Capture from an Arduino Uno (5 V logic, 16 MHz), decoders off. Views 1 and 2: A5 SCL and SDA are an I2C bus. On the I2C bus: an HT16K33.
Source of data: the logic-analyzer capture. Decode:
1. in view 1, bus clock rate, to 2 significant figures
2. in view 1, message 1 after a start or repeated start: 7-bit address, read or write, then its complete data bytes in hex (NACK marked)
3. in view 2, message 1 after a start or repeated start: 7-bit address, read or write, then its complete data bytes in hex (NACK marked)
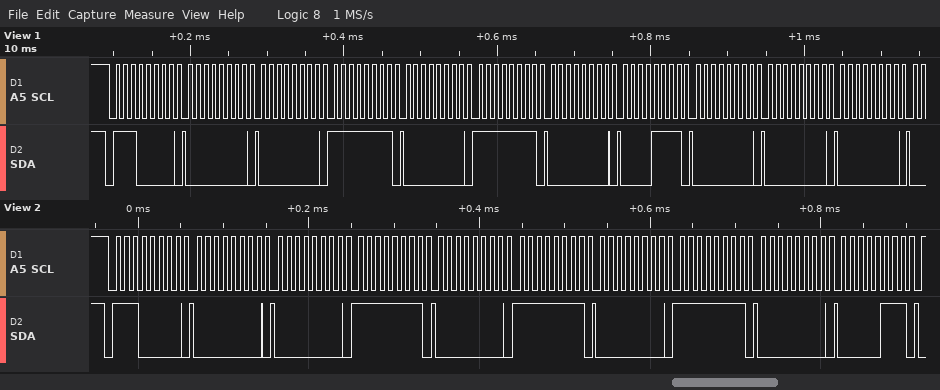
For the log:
100 kHz
0x70 write: 00 00 FF 00 FF 00 0F 00 00 00
0x70 write: 00 00 FF 00 FF 00 FF 00 07
